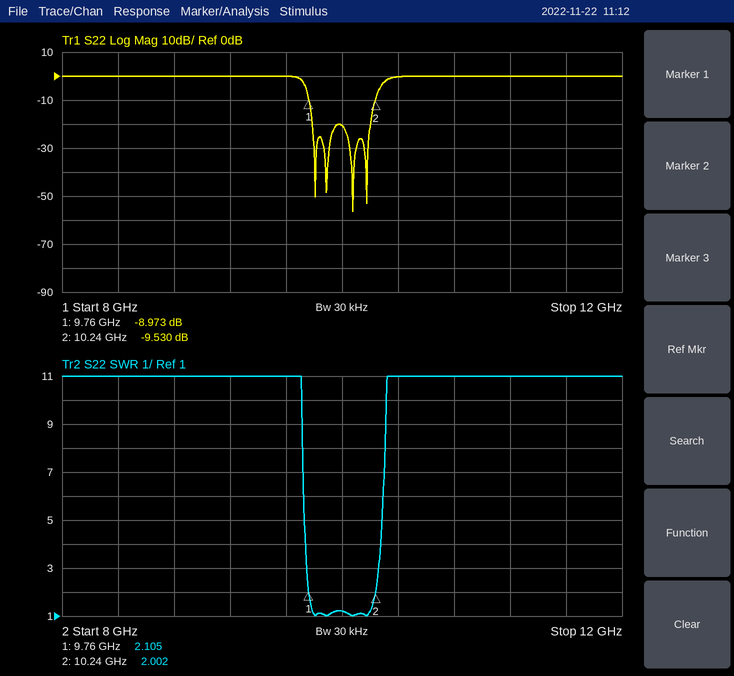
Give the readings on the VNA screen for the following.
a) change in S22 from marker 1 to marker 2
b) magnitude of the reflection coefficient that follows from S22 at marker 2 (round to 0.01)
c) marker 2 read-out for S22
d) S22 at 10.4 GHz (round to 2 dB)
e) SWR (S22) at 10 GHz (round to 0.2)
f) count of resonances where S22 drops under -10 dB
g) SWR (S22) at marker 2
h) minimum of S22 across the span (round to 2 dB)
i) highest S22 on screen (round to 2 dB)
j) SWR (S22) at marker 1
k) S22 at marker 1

-0.557 dB
0.33
-9.530 dB
0 dB
1.2
4
2.002
-56 dB
0 dB
2.105
-8.973 dB
